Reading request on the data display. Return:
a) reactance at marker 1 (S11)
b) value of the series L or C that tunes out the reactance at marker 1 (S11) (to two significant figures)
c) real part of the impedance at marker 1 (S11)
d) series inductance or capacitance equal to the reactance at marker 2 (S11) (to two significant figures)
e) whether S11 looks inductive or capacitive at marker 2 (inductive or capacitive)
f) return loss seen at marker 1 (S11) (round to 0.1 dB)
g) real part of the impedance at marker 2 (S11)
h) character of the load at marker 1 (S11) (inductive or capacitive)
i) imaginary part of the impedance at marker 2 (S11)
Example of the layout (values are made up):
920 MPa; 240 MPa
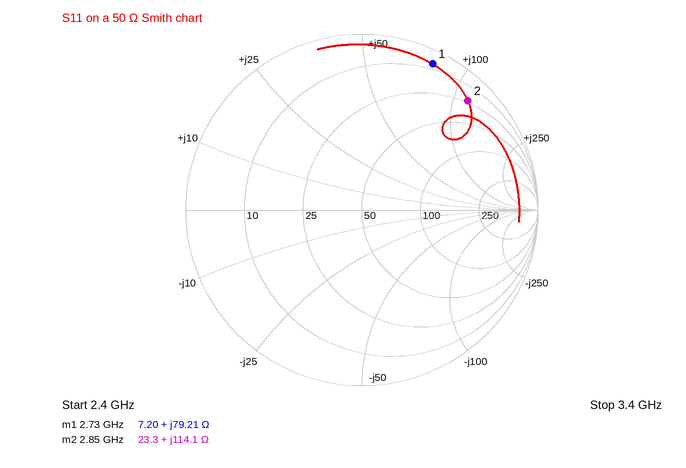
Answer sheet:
+79.21 Ω; 740 fF; 7.20 Ω; 6.4 nH; inductive; 0.7 dB; 23.3 Ω; inductive; +114.1 Ω
